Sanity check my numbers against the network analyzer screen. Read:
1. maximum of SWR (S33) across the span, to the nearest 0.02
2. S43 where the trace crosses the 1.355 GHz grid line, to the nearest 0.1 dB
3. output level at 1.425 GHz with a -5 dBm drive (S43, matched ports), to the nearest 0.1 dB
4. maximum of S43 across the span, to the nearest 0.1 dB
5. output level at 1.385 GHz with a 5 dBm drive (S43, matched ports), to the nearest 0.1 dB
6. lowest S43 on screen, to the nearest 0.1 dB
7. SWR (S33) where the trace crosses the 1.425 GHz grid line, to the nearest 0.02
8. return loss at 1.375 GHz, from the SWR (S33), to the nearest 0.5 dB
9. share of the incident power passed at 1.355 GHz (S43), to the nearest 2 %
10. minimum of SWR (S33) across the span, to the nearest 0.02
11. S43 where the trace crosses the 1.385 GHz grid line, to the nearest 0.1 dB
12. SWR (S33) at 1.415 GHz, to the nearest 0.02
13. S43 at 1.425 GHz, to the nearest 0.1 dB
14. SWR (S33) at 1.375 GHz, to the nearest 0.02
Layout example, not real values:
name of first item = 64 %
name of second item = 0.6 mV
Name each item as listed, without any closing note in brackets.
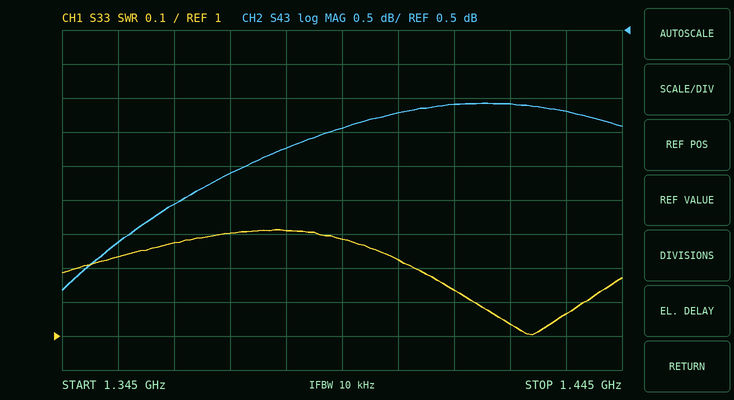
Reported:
maximum of SWR (S33) across the span, to the nearest 0.02 = 1.32
S43 where the trace crosses the 1.355 GHz grid line, to the nearest 0.1 dB = -2.6 dB
output level at 1.425 GHz with a -5 dBm drive (S43, matched ports), to the nearest 0.1 dB = -5.6 dBm
maximum of S43 across the span, to the nearest 0.1 dB = -0.6 dB
output level at 1.385 GHz with a 5 dBm drive (S43, matched ports), to the nearest 0.1 dB = 3.8 dBm
lowest S43 on screen, to the nearest 0.1 dB = -3.3 dB
SWR (S33) where the trace crosses the 1.425 GHz grid line, to the nearest 0.02 = 1.04
return loss at 1.375 GHz, from the SWR (S33), to the nearest 0.5 dB = 17.5 dB
share of the incident power passed at 1.355 GHz (S43), to the nearest 2 % = 54 %
minimum of SWR (S33) across the span, to the nearest 0.02 = 1.00
S43 where the trace crosses the 1.385 GHz grid line, to the nearest 0.1 dB = -1.2 dB
SWR (S33) at 1.415 GHz, to the nearest 0.02 = 1.14
S43 at 1.425 GHz, to the nearest 0.1 dB = -0.6 dB
SWR (S33) at 1.375 GHz, to the nearest 0.02 = 1.30
